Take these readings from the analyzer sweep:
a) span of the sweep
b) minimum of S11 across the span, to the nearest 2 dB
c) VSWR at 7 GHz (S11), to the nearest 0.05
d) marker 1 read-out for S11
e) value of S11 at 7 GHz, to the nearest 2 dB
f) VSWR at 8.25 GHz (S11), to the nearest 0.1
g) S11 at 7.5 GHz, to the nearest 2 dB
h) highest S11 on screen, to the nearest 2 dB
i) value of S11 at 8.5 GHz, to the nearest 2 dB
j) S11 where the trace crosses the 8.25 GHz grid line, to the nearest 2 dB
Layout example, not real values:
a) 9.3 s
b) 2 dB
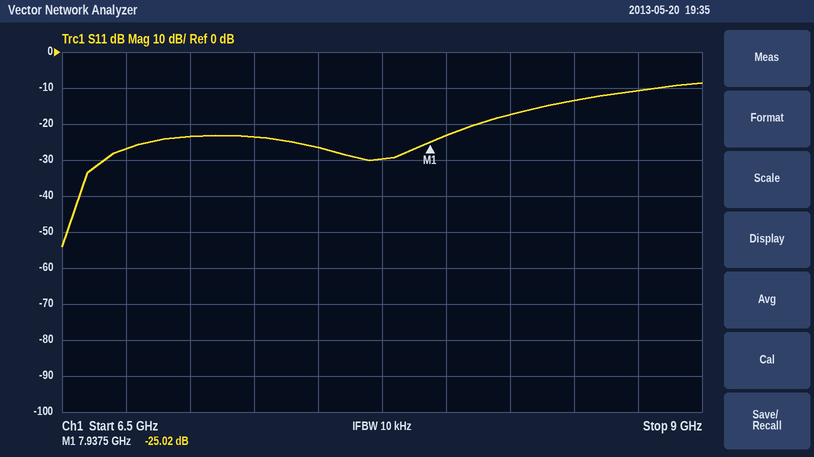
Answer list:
a) 2.5 GHz
b) -54 dB
c) 1.15
d) -25.02 dB
e) -24 dB
f) 1.3
g) -26 dB
h) -8 dB
i) -14 dB
j) -18 dB
